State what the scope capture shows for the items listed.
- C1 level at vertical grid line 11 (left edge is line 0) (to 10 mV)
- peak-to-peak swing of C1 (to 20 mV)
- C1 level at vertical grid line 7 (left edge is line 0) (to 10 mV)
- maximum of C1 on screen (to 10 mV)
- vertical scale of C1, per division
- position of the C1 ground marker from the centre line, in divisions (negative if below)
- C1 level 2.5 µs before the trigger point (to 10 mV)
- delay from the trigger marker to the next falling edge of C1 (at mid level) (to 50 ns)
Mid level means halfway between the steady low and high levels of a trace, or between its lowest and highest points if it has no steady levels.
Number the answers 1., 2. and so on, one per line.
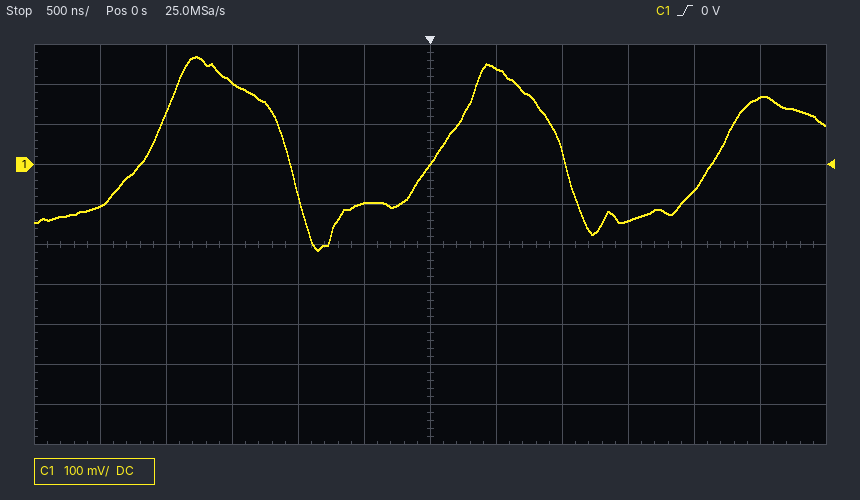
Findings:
1. 170 mV
2. 480 mV
3. 240 mV
4. 270 mV
5. 100 mV
6. +2.0 div
7. -100 mV
8. 1.00 µs
